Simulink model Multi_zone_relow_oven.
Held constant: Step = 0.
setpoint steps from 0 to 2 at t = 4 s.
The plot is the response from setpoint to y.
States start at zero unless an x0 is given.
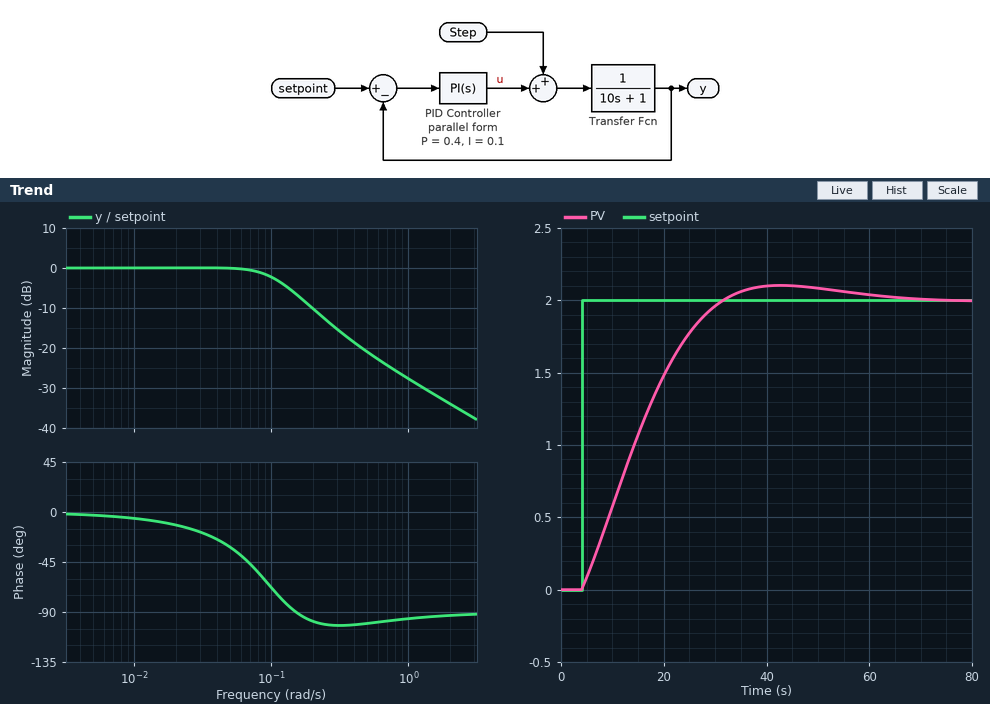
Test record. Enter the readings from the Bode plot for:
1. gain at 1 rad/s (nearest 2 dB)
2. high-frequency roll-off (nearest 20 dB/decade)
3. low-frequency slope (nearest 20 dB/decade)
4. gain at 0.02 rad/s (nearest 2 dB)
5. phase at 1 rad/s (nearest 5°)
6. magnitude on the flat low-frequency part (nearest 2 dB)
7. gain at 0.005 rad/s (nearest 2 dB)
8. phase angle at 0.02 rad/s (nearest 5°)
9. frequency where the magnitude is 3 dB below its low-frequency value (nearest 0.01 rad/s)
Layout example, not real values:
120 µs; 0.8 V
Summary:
-28 dB; -20 dB/decade; 0 dB/decade; 0 dB; -95°; 0 dB; 0 dB; -10°; 0.11 rad/s
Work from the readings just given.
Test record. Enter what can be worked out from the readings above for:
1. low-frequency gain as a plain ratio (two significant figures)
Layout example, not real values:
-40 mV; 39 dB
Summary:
1.0
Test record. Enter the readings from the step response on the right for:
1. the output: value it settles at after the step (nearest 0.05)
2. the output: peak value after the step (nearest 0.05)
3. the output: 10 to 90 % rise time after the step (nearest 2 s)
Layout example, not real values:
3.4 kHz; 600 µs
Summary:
2.00; 2.10; 20 s
